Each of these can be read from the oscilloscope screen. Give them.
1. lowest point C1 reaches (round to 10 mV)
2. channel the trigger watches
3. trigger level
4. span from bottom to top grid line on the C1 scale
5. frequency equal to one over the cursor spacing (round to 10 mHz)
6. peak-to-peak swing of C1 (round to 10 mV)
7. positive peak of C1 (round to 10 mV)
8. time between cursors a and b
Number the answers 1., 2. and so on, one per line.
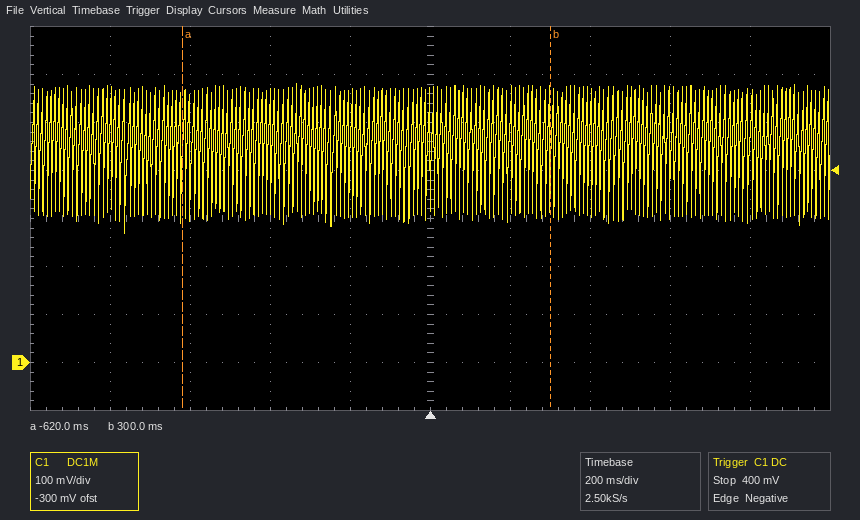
1. 270 mV
2. C1
3. 400 mV
4. 800 mV
5. 1.09 Hz
6. 310 mV
7. 580 mV
8. 920 ms
